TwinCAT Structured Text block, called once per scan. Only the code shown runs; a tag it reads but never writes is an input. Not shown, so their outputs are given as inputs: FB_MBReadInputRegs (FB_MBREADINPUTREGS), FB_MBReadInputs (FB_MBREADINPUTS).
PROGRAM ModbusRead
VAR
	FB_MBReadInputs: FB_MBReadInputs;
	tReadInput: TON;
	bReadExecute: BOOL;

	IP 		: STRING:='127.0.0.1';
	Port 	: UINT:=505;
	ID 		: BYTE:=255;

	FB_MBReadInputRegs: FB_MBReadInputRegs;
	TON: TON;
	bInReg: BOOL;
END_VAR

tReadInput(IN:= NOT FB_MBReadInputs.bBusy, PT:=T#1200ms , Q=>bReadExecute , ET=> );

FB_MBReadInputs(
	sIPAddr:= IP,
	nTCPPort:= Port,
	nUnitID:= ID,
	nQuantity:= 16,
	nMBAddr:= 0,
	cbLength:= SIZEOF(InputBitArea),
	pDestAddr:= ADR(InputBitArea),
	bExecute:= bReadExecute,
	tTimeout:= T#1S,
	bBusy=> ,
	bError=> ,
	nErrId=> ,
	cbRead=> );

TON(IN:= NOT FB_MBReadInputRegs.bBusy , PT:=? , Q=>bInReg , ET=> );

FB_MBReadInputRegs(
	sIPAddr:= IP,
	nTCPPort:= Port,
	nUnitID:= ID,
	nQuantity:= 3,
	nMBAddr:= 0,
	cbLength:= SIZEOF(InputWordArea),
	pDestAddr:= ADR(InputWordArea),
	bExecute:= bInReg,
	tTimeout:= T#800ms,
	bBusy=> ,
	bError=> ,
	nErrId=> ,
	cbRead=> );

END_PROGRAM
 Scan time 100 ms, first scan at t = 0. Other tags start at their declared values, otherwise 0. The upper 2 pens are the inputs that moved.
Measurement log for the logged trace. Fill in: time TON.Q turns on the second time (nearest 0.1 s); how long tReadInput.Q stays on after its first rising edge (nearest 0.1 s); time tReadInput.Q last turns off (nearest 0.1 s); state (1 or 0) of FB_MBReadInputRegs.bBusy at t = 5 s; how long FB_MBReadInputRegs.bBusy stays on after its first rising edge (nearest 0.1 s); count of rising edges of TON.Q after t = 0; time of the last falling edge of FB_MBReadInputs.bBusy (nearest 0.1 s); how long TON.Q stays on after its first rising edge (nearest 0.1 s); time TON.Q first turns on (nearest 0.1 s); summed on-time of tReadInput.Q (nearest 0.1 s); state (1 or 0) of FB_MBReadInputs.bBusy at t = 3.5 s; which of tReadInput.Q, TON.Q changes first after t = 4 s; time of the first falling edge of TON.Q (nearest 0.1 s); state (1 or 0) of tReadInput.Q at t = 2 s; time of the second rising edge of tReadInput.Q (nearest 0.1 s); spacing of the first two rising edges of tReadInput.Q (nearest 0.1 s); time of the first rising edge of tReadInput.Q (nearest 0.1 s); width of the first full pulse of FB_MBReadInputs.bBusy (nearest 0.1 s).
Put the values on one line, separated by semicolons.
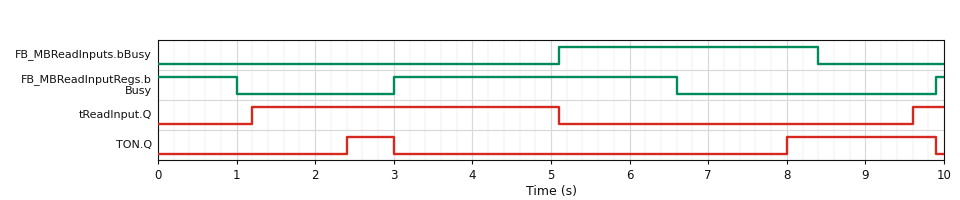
8.0 s; 3.9 s; 5.1 s; 1; 3.6 s; 2; 8.4 s; 0.6 s; 2.4 s; 4.3 s; 0; tReadInput.Q; 3.0 s; 1; 9.6 s; 8.4 s; 1.2 s; 3.3 s
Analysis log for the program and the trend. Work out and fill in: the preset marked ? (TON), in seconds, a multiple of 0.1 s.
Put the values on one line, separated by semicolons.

1.4 s
